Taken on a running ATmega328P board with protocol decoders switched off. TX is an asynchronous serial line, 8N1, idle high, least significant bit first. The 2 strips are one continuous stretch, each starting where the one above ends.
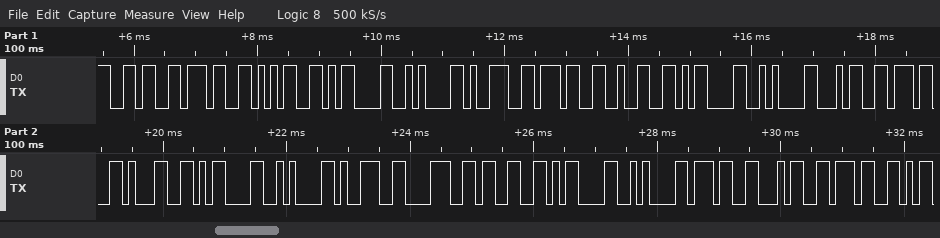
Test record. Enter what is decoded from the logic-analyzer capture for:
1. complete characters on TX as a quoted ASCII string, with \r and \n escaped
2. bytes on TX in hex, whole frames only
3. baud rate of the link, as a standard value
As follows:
"675\r\n972\r\n471\r\n983\r\n747"
36 37 35 0D 0A 39 37 32 0D 0A 34 37 31 0D 0A 39 38 33 0D 0A 37 34 37
9600 baud
